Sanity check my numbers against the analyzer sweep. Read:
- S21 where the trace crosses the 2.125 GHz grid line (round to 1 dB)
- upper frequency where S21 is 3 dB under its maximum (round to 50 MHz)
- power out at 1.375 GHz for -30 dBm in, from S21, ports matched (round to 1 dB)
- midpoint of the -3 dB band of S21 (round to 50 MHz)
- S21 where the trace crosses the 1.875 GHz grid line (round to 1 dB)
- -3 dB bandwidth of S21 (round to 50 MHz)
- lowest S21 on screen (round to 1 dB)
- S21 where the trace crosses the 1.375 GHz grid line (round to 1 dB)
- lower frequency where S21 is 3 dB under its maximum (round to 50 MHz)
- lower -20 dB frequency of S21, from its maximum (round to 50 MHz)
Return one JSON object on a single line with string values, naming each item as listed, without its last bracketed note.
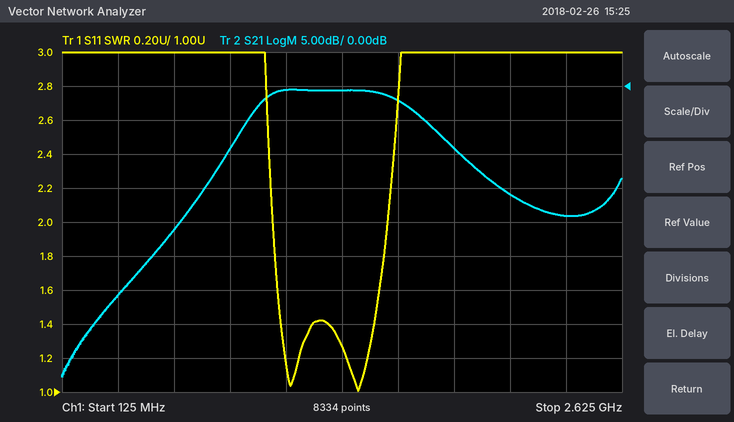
{"S21 where the trace crosses the 2.125 GHz grid line": "-16 dB", "upper frequency where S21 is 3 dB under its maximum": "1.70 GHz", "power out at 1.375 GHz for -30 dBm in, from S21, ports matched": "-31 dBm", "midpoint of the -3 dB band of S21": "1.35 GHz", "S21 where the trace crosses the 1.875 GHz grid line": "-9 dB", "-3 dB bandwidth of S21": "700 MHz", "lowest S21 on screen": "-43 dB", "S21 where the trace crosses the 1.375 GHz grid line": "-1 dB", "lower frequency where S21 is 3 dB under its maximum": "1.00 GHz", "lower -20 dB frequency of S21, from its maximum": "650 MHz"}
